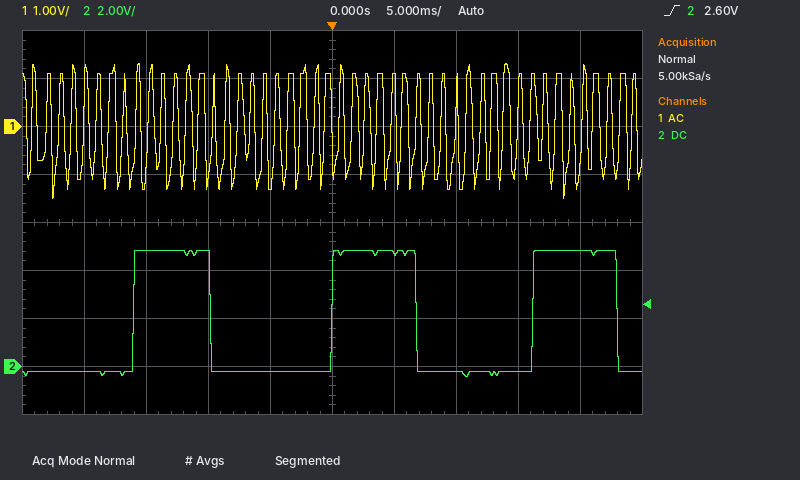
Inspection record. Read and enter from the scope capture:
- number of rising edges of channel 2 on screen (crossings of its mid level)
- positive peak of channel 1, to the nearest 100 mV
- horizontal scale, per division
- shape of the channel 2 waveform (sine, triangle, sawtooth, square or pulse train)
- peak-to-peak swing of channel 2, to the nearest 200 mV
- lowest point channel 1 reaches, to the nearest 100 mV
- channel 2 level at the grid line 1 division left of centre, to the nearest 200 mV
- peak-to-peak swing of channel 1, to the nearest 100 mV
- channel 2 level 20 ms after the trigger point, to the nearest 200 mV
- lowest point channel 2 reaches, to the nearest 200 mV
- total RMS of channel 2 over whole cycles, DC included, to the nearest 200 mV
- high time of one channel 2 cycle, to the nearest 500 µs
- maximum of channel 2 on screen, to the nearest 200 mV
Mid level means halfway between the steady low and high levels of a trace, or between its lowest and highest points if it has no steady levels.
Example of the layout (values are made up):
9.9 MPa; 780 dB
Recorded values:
3; 1.3 V; 5 ms; pulse train; 5.2 V; -1.5 V; -200 mV; 2.8 V; 4.8 V; -400 mV; 3.0 V; 6.5 ms; 4.8 V
